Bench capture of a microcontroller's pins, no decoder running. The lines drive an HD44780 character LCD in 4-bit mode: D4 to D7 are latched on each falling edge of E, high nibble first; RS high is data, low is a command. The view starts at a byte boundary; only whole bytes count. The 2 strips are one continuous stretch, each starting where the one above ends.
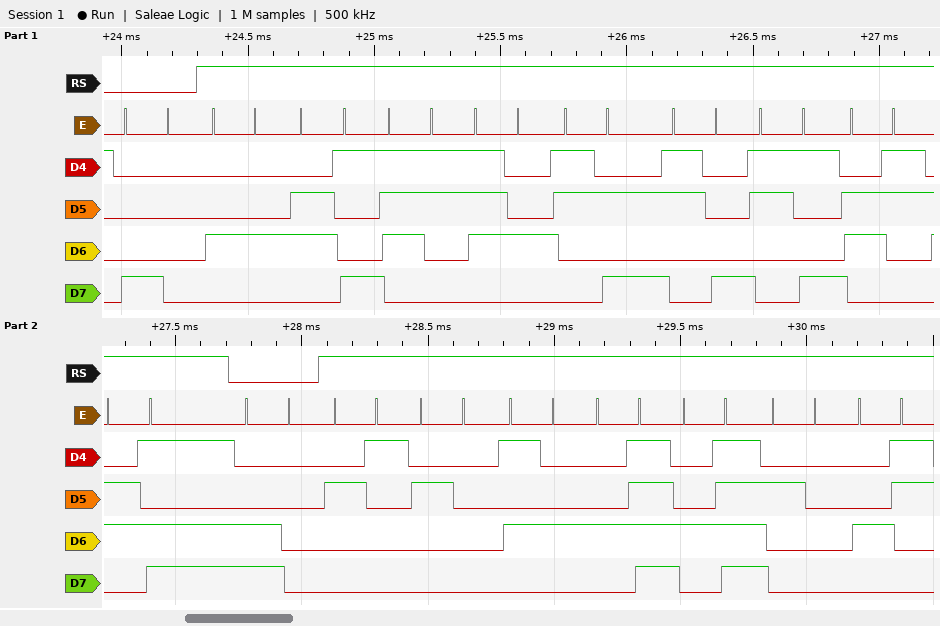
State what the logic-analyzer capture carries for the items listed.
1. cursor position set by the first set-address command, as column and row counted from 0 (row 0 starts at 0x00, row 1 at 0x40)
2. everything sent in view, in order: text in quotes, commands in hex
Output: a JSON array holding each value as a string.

["column 0, row 0", "0x80 \"Dist:89cm\" 0xC0 \"! TOO C\""]
